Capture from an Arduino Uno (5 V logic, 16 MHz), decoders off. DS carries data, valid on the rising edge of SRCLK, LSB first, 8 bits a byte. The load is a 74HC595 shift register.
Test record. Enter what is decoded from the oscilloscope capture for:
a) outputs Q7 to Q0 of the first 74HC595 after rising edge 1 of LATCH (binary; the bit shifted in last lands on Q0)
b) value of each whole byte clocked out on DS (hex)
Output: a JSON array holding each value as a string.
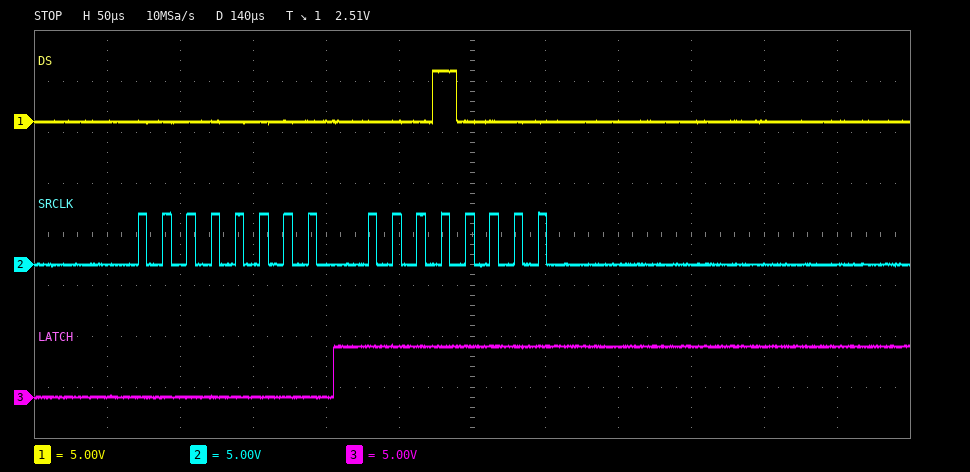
["00000000", "00 08"]
